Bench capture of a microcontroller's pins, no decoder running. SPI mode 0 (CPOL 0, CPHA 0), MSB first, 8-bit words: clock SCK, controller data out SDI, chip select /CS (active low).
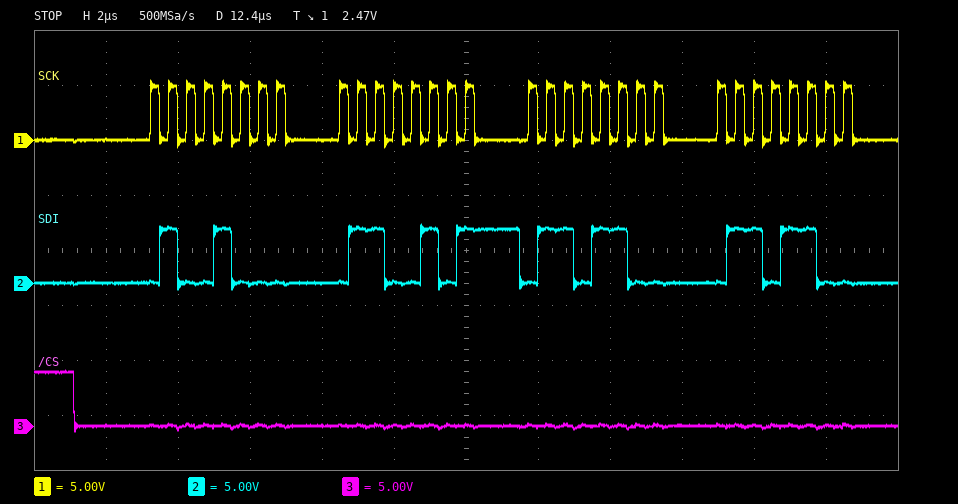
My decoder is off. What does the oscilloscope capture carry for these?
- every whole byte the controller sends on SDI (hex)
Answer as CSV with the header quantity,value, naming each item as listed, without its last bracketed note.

quantity,value
every whole byte the controller sends on SDI,0x48 0x65 0x6C 0x6C
